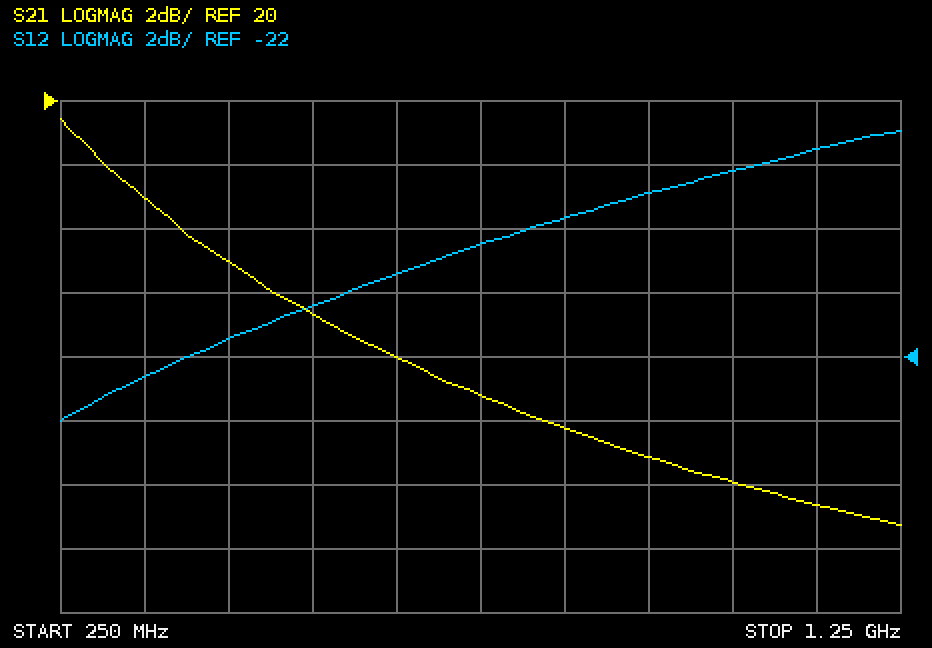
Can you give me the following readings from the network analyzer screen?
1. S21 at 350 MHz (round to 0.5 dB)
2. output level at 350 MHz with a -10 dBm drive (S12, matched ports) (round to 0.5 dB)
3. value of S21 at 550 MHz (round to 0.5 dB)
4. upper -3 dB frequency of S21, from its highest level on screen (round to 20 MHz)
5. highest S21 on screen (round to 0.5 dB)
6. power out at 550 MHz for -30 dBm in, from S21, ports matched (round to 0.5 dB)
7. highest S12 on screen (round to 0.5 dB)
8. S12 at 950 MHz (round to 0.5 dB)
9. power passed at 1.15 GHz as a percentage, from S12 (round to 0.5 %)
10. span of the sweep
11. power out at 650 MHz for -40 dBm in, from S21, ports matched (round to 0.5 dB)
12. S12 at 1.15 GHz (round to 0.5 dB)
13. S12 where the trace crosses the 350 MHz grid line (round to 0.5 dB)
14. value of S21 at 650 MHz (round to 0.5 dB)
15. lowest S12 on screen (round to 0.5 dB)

17.0 dB
-32.5 dBm
13.5 dB
380 MHz
19.5 dB
-16.5 dBm
-15.0 dB
-17.0 dB
3.0 %
1 GHz
-28.0 dBm
-15.5 dB
-22.5 dB
12.0 dB
-24.0 dB
